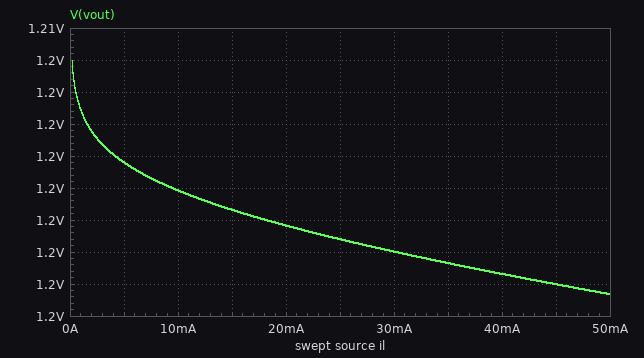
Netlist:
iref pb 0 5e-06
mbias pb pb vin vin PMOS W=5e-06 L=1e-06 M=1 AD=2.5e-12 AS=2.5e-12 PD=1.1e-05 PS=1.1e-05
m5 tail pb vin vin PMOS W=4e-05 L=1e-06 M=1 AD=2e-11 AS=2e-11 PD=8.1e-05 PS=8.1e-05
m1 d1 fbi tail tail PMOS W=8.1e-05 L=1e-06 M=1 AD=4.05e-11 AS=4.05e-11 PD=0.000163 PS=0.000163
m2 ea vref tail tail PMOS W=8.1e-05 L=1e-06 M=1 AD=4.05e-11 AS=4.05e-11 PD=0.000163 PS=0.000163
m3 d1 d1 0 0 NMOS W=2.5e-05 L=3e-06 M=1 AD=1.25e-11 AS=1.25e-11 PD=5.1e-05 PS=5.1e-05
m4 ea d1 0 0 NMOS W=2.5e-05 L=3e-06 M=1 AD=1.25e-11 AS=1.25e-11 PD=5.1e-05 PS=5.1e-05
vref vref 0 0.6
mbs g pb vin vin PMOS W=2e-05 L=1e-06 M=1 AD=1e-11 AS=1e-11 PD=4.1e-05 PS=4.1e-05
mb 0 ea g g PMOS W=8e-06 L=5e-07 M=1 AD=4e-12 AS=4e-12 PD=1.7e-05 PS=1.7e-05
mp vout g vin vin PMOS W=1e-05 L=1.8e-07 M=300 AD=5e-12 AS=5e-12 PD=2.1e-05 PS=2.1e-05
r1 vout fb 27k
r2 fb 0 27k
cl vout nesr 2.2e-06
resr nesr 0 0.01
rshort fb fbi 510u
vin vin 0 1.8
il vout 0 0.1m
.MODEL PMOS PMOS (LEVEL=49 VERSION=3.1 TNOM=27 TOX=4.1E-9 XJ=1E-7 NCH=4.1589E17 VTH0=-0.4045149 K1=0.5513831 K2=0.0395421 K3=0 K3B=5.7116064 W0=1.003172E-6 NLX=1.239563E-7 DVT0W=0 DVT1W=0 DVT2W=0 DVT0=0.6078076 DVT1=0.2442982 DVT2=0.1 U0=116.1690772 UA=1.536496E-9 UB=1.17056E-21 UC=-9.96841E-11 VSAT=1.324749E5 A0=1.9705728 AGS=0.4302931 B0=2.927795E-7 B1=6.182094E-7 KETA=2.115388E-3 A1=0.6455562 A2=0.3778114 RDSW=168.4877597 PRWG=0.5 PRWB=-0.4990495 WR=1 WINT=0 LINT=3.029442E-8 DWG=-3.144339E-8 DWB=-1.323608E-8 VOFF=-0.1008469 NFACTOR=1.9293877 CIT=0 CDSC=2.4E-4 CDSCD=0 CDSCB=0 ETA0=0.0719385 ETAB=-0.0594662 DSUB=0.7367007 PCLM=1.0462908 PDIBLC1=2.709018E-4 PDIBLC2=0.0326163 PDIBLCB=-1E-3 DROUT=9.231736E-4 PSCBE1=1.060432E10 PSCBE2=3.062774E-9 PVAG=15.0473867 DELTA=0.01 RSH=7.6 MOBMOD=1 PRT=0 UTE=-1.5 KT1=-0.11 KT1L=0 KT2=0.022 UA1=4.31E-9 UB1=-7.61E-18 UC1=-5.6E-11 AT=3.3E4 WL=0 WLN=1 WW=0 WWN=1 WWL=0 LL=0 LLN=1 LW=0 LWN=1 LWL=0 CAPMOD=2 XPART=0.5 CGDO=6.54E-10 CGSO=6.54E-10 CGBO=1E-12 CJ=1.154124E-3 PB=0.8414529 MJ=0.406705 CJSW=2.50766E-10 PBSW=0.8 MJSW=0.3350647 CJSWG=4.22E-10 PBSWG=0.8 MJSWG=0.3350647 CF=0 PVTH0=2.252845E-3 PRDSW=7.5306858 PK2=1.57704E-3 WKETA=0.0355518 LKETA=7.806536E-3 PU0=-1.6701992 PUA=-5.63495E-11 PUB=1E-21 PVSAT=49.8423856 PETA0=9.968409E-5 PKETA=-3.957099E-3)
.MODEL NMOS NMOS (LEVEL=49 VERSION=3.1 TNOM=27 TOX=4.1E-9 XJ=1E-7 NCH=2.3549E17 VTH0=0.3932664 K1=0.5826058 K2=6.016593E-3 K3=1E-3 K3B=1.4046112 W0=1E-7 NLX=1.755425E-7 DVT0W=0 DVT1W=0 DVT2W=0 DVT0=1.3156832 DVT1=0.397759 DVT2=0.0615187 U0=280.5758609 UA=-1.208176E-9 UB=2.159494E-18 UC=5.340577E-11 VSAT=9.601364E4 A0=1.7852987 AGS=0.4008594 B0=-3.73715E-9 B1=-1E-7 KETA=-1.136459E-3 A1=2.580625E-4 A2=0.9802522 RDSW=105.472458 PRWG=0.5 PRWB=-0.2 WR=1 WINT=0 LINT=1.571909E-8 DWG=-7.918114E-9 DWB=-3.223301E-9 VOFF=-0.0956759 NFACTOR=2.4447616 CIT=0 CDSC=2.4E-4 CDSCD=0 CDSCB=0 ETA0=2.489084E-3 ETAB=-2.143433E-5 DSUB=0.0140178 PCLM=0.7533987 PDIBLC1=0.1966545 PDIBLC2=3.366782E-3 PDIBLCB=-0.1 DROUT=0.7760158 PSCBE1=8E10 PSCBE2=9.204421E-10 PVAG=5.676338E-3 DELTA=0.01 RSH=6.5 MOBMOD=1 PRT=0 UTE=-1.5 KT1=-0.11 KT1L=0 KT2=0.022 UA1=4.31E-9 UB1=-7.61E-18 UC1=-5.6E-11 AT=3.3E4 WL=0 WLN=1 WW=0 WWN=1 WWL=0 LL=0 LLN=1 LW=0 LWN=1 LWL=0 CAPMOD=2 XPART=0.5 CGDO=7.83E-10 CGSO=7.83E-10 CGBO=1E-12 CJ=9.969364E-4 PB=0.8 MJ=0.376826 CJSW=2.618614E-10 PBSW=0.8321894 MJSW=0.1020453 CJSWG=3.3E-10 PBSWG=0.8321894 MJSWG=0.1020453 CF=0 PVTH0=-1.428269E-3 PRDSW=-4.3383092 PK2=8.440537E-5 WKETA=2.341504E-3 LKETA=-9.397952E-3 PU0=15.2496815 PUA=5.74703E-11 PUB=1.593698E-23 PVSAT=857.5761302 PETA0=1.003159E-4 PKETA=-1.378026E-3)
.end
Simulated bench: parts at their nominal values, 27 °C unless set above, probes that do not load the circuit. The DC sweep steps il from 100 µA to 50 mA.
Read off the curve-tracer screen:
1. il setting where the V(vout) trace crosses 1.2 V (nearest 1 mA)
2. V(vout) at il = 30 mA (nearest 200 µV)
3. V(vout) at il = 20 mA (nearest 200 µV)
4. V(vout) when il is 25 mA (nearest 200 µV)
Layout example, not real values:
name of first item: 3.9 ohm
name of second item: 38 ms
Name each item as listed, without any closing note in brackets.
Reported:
il setting where the V(vout) trace crosses 1.2 V: 4 mA
V(vout) at il = 30 mA: 1.1980 V
V(vout) at il = 20 mA: 1.1988 V
V(vout) when il is 25 mA: 1.1984 V
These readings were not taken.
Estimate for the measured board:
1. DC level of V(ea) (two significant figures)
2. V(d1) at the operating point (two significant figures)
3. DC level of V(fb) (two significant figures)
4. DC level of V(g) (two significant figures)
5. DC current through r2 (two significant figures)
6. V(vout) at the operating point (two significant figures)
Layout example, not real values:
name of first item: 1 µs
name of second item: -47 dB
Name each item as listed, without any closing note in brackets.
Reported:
DC level of V(ea): 780 mV
V(d1) at the operating point: 560 mV
DC level of V(fb): 600 mV
DC level of V(g): 1.4 V
DC current through r2: 22 µA
V(vout) at the operating point: 1.2 V
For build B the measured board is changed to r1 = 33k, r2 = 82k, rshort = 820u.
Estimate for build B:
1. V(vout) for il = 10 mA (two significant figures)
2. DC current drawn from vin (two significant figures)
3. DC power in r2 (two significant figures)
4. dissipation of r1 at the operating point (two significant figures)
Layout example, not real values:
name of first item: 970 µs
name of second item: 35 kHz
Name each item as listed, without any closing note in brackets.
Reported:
V(vout) for il = 10 mA: 840 mV
DC current drawn from vin: 170 µA
DC power in r2: 4.4 µW
dissipation of r1 at the operating point: 1.8 µW
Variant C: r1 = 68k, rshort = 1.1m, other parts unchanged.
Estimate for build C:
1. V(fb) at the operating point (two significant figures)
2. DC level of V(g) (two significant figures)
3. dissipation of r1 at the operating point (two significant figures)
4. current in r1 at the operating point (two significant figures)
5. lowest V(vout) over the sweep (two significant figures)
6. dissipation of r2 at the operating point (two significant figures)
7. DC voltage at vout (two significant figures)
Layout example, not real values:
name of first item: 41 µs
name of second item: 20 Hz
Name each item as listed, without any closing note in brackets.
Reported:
V(fb) at the operating point: 510 mV
DC level of V(g): 670 mV
dissipation of r1 at the operating point: 24 µW
current in r1 at the operating point: 19 µA
lowest V(vout) over the sweep: 1.7 V
dissipation of r2 at the operating point: 9.7 µW
DC voltage at vout: 1.8 V
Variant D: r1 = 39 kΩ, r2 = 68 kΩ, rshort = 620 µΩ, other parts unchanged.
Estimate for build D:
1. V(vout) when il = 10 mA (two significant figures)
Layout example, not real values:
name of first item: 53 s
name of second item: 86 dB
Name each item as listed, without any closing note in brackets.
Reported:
V(vout) when il = 10 mA: 940 mV
